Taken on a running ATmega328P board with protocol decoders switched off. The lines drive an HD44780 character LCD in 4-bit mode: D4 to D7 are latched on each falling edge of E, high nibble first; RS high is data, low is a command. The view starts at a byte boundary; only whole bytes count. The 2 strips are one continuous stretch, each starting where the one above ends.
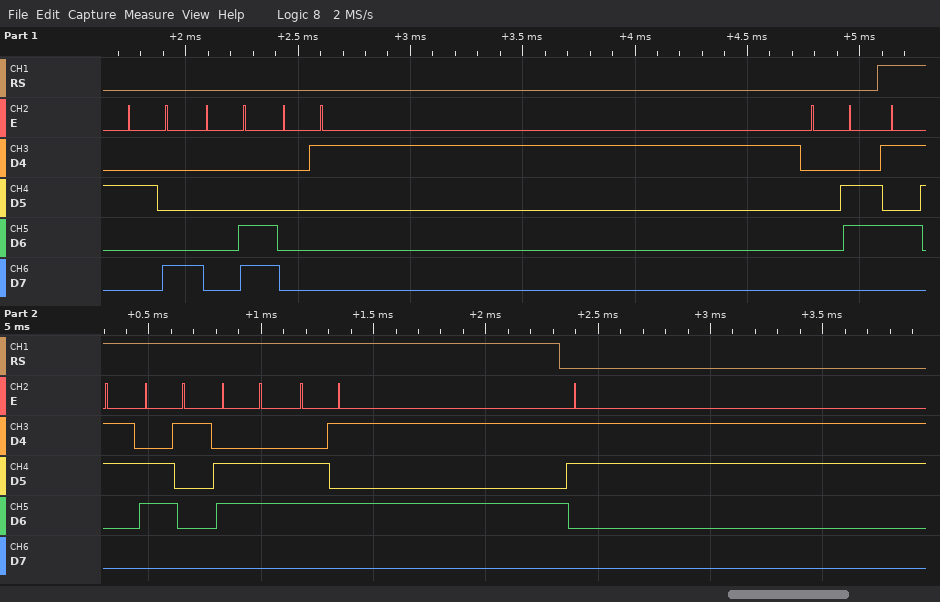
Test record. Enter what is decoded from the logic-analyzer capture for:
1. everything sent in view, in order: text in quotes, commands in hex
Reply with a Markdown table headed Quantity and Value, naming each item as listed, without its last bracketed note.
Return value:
| Quantity | Value |
|---|---|
| everything sent in view, in order: text in quotes, commands in hex | 0x28 0x0C 0x01 0x06 "Safe" |
